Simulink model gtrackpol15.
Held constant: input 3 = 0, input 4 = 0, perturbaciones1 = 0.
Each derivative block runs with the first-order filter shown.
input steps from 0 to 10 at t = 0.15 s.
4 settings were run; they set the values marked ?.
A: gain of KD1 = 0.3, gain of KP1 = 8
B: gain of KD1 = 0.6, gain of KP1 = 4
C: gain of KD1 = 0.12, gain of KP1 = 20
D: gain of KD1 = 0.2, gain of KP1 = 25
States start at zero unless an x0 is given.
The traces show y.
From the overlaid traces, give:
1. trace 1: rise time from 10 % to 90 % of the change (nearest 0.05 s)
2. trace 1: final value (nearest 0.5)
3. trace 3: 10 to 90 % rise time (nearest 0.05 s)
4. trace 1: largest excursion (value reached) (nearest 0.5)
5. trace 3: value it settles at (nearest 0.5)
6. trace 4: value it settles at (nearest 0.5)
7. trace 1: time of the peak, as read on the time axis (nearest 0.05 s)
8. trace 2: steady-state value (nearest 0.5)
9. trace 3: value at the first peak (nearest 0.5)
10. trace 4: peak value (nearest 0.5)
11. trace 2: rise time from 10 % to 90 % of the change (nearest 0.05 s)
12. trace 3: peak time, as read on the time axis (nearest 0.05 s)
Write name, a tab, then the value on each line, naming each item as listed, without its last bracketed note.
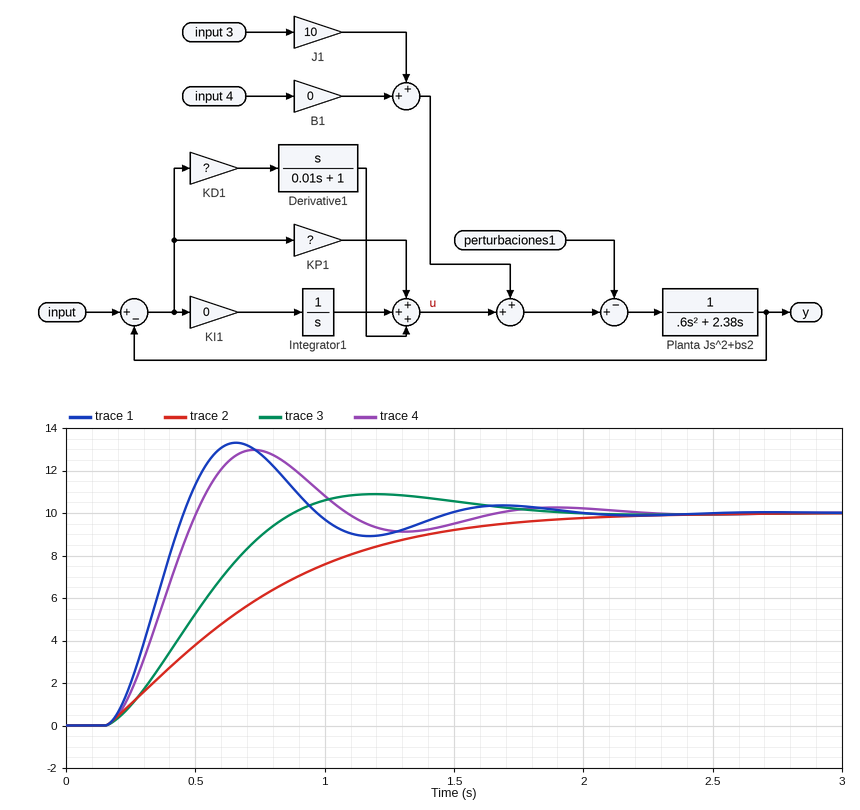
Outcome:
trace 1: rise time from 10 % to 90 % of the change	0.20 s
trace 1: final value	10.0
trace 3: 10 to 90 % rise time	0.50 s
trace 1: largest excursion (value reached)	13.5
trace 3: value it settles at	10.0
trace 4: value it settles at	10.0
trace 1: time of the peak, as read on the time axis	0.65 s
trace 2: steady-state value	10.0
trace 3: value at the first peak	11.0
trace 4: peak value	13.0
trace 2: rise time from 10 % to 90 % of the change	1.15 s
trace 3: peak time, as read on the time axis	1.20 s
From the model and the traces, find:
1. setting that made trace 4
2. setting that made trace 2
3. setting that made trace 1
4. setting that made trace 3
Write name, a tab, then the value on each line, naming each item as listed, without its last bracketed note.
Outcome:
setting that made trace 4	C
setting that made trace 2	B
setting that made trace 1	D
setting that made trace 3	A
